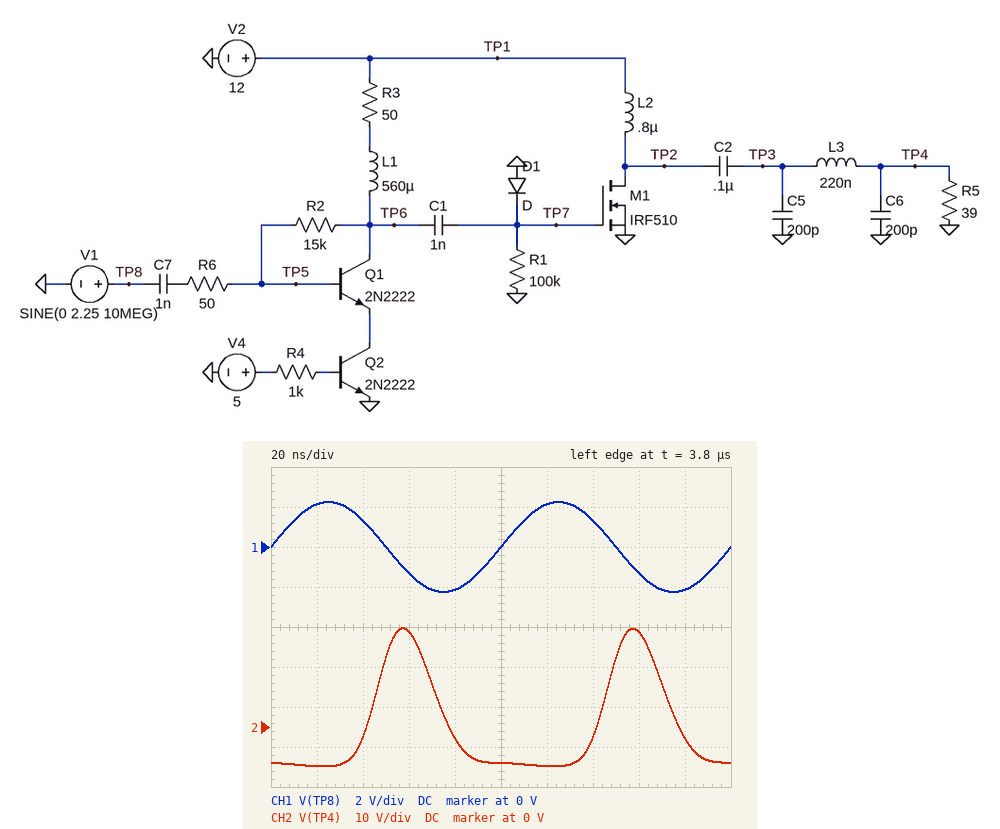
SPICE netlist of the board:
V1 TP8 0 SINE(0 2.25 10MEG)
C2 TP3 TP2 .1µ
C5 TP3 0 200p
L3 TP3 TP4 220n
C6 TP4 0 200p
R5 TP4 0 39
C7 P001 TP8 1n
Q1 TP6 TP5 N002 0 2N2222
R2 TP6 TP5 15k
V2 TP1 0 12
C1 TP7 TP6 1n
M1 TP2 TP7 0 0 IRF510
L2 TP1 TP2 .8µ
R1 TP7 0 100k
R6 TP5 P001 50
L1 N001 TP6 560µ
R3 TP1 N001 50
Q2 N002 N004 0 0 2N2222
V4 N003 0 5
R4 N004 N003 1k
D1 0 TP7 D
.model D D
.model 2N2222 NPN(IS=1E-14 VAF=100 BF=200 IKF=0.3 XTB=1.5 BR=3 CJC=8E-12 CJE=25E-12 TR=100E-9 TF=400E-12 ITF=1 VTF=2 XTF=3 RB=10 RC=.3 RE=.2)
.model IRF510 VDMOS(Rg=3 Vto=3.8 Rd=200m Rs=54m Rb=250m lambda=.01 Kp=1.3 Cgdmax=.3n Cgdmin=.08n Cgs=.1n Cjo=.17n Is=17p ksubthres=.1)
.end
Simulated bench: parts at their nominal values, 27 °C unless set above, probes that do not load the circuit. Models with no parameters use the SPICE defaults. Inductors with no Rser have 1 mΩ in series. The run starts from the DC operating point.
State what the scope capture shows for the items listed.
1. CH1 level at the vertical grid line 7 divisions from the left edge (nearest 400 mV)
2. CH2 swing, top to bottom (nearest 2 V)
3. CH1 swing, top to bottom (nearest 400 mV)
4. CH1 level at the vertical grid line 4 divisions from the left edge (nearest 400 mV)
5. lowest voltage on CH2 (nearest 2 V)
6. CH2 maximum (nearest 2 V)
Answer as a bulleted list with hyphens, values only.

- 1.2 V
- 34 V
- 4.4 V
- -2.0 V
- -10 V
- 24 V
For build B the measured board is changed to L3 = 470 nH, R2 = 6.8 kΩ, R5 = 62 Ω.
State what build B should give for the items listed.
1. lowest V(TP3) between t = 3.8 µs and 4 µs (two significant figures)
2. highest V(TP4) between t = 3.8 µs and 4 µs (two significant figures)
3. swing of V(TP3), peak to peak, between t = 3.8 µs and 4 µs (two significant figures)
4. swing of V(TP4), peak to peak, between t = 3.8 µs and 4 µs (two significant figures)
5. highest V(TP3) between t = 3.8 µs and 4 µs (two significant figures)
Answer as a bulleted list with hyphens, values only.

- -12 V
- 26 V
- 34 V
- 43 V
- 22 V
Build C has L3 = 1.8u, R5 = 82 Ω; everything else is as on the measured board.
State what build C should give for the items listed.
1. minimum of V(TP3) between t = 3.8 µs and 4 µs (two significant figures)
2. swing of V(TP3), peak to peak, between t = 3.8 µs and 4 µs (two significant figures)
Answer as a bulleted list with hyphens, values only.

- -6.8 V
- 27 V
